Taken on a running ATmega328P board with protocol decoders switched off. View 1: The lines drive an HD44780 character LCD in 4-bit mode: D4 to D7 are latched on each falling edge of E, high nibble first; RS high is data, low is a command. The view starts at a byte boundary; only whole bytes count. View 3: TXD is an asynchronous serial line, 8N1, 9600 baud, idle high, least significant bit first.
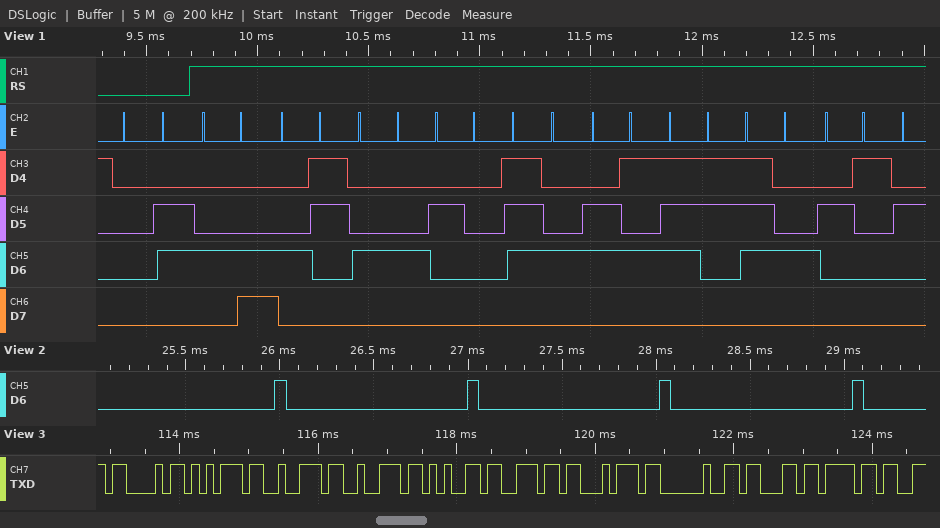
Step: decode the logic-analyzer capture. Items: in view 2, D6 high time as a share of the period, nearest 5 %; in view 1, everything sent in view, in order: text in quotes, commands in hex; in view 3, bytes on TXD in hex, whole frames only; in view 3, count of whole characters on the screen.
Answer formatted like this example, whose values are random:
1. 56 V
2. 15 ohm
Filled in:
1. 5 %
2. 0x06 "LCD test!"
3. 43 75 72 72 65 6E 74 20 63 6F
4. 10
